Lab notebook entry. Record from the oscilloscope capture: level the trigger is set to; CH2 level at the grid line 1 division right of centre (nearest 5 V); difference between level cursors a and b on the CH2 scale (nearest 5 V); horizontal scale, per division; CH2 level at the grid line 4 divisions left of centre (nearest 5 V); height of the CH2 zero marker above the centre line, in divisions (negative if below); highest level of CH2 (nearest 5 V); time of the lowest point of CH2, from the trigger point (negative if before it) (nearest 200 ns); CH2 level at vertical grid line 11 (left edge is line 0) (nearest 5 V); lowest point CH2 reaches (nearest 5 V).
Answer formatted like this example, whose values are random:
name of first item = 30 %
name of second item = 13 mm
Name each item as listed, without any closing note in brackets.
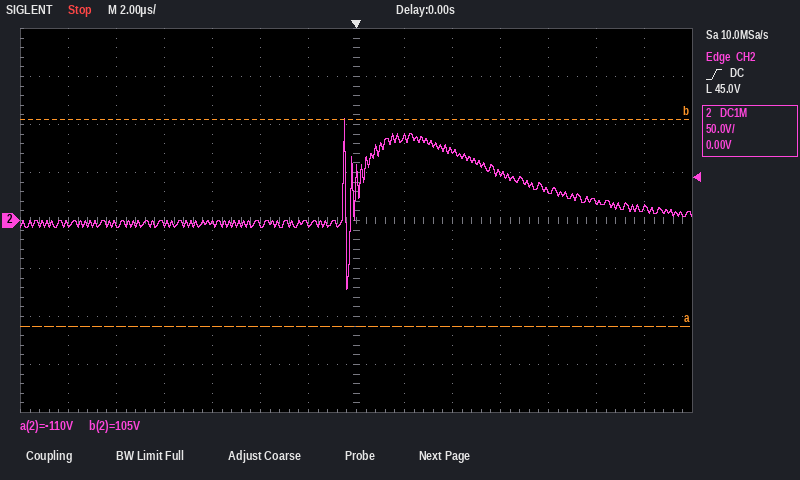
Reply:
level the trigger is set to = 45.0 V
CH2 level at the grid line 1 division right of centre = 85 V
difference between level cursors a and b on the CH2 scale = 215 V
horizontal scale, per division = 2 µs
CH2 level at the grid line 4 divisions left of centre = -5 V
height of the CH2 zero marker above the centre line, in divisions = 0.0 div
highest level of CH2 = 105 V
time of the lowest point of CH2, from the trigger point (negative if before it) = -400 ns
CH2 level at vertical grid line 11 (left edge is line 0) = 30 V
lowest point CH2 reaches = -70 V
